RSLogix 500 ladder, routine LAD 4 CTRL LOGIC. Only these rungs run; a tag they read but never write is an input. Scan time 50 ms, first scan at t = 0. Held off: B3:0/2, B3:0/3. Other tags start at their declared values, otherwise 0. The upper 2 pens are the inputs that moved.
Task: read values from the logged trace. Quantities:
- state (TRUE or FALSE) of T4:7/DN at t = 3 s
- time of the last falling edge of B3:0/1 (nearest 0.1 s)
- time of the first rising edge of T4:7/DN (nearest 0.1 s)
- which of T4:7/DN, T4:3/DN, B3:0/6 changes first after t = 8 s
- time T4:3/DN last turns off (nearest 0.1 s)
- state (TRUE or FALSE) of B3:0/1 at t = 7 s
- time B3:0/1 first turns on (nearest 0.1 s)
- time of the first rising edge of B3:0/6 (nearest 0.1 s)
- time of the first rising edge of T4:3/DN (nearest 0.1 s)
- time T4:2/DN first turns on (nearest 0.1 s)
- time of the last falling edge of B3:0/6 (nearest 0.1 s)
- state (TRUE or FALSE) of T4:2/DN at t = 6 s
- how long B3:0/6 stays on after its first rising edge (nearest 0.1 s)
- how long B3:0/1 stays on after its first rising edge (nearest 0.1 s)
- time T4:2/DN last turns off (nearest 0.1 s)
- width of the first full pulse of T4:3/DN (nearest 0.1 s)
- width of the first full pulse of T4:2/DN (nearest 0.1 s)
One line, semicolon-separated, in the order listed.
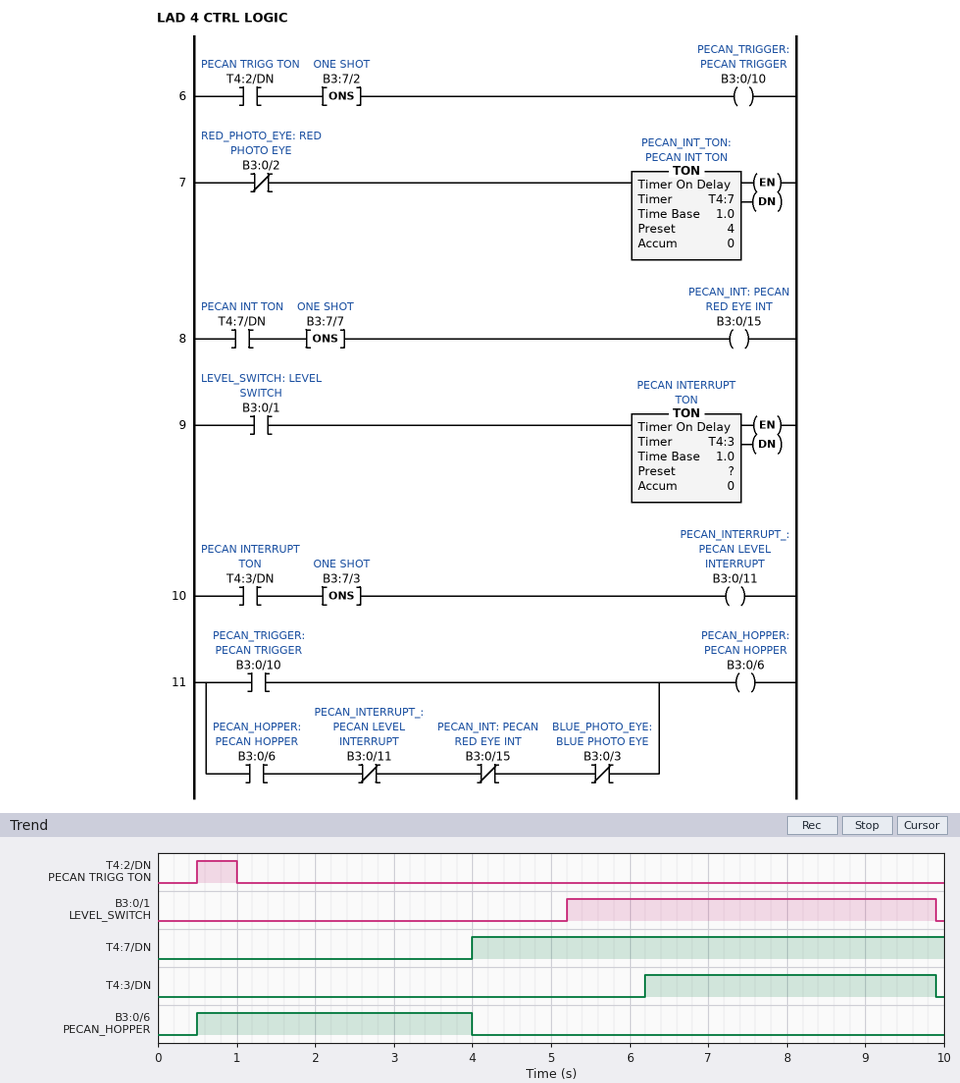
FALSE; 9.9 s; 4.0 s; T4:3/DN; 9.9 s; TRUE; 5.2 s; 0.5 s; 6.2 s; 0.5 s; 4.0 s; FALSE; 3.5 s; 4.7 s; 1.0 s; 3.7 s; 0.5 s
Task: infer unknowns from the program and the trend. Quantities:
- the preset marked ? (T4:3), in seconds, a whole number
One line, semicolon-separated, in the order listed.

1 s
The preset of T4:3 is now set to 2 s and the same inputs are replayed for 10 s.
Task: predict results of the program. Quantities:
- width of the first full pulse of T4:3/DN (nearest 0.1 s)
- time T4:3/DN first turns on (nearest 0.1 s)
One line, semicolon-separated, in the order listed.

2.7 s; 7.2 s
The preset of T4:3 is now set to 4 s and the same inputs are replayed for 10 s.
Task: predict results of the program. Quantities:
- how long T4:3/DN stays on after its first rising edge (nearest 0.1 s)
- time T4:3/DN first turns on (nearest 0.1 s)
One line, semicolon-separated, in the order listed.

0.7 s; 9.2 s
